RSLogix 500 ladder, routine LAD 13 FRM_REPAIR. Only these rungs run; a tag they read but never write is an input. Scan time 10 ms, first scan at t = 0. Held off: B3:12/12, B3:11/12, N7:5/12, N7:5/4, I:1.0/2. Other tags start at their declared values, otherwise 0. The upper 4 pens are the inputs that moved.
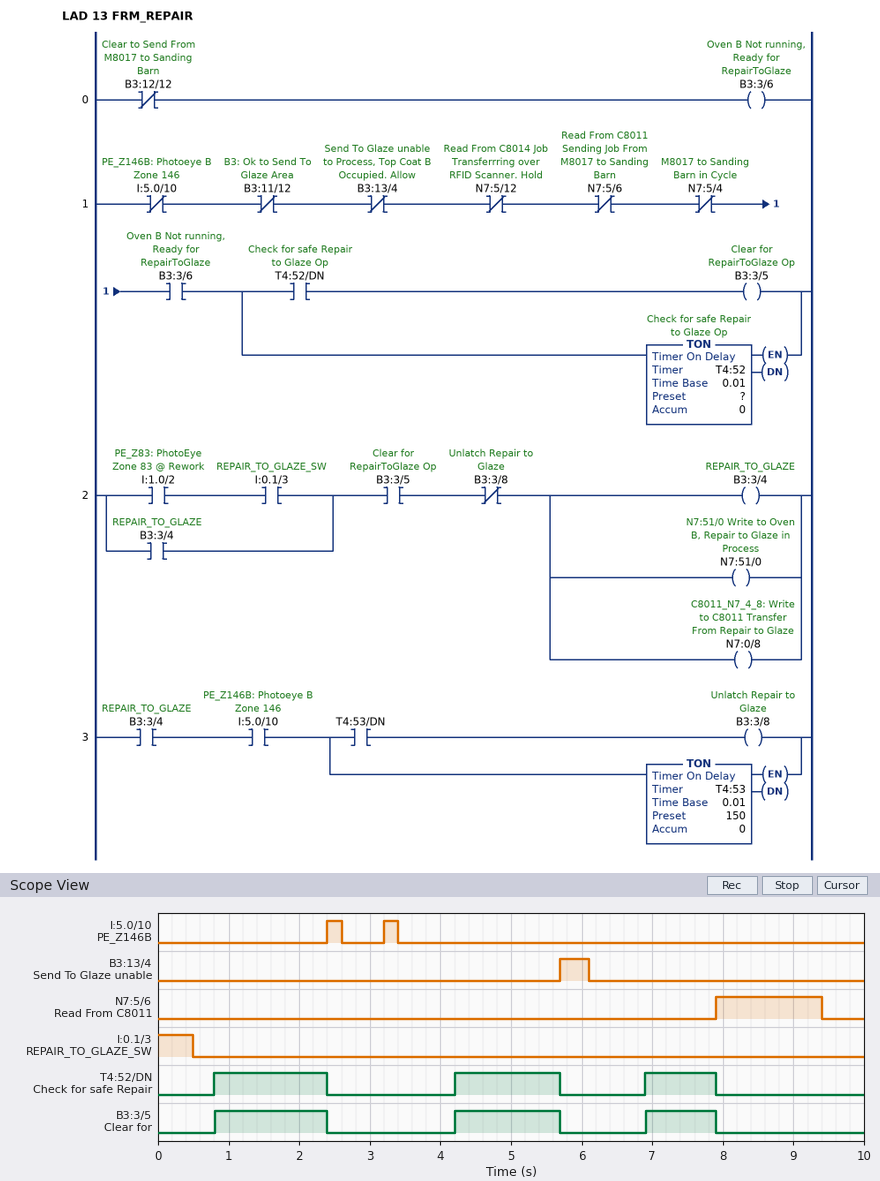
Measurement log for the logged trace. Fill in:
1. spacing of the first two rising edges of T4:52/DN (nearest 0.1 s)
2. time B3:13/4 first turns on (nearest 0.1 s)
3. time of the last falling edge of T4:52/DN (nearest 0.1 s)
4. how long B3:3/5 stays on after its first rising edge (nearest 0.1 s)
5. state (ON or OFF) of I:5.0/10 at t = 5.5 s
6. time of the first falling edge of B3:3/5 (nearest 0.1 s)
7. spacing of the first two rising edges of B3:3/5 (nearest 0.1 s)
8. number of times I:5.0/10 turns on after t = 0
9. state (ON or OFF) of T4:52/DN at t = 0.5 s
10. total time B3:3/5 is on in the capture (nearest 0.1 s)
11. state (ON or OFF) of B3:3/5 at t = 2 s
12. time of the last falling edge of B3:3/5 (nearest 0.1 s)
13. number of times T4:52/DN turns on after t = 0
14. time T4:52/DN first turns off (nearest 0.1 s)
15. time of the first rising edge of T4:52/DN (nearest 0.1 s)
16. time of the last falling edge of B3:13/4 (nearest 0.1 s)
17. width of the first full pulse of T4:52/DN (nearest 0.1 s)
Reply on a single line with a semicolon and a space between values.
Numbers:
3.4 s; 5.7 s; 7.9 s; 1.6 s; OFF; 2.4 s; 3.4 s; 2; OFF; 4.1 s; ON; 7.9 s; 3; 2.4 s; 0.8 s; 6.1 s; 1.6 s
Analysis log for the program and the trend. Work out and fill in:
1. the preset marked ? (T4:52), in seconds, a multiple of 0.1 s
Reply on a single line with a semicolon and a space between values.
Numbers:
0.8 s
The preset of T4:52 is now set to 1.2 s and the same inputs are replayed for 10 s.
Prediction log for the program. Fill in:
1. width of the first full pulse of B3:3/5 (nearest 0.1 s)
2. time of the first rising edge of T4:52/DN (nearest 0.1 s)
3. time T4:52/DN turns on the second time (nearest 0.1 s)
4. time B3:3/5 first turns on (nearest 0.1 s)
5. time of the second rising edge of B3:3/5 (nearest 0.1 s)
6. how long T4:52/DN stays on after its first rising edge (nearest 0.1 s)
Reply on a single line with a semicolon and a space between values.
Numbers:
1.2 s; 1.2 s; 4.6 s; 1.2 s; 4.6 s; 1.2 s
